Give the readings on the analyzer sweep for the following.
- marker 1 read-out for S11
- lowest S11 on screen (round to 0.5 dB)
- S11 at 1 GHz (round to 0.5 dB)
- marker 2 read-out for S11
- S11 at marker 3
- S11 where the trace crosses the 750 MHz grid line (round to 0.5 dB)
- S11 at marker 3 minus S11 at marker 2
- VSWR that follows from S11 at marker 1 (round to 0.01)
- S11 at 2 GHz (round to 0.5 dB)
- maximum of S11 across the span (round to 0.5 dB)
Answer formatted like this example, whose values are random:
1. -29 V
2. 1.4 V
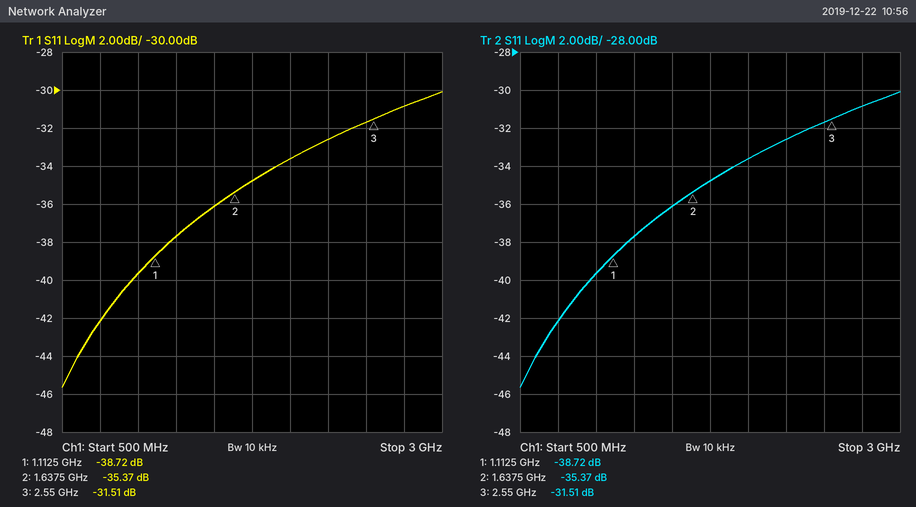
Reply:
1. -38.72 dB
2. -45.5 dB
3. -39.5 dB
4. -35.37 dB
5. -31.51 dB
6. -42.0 dB
7. 3.86 dB
8. 1.02
9. -33.5 dB
10. -30.0 dB
